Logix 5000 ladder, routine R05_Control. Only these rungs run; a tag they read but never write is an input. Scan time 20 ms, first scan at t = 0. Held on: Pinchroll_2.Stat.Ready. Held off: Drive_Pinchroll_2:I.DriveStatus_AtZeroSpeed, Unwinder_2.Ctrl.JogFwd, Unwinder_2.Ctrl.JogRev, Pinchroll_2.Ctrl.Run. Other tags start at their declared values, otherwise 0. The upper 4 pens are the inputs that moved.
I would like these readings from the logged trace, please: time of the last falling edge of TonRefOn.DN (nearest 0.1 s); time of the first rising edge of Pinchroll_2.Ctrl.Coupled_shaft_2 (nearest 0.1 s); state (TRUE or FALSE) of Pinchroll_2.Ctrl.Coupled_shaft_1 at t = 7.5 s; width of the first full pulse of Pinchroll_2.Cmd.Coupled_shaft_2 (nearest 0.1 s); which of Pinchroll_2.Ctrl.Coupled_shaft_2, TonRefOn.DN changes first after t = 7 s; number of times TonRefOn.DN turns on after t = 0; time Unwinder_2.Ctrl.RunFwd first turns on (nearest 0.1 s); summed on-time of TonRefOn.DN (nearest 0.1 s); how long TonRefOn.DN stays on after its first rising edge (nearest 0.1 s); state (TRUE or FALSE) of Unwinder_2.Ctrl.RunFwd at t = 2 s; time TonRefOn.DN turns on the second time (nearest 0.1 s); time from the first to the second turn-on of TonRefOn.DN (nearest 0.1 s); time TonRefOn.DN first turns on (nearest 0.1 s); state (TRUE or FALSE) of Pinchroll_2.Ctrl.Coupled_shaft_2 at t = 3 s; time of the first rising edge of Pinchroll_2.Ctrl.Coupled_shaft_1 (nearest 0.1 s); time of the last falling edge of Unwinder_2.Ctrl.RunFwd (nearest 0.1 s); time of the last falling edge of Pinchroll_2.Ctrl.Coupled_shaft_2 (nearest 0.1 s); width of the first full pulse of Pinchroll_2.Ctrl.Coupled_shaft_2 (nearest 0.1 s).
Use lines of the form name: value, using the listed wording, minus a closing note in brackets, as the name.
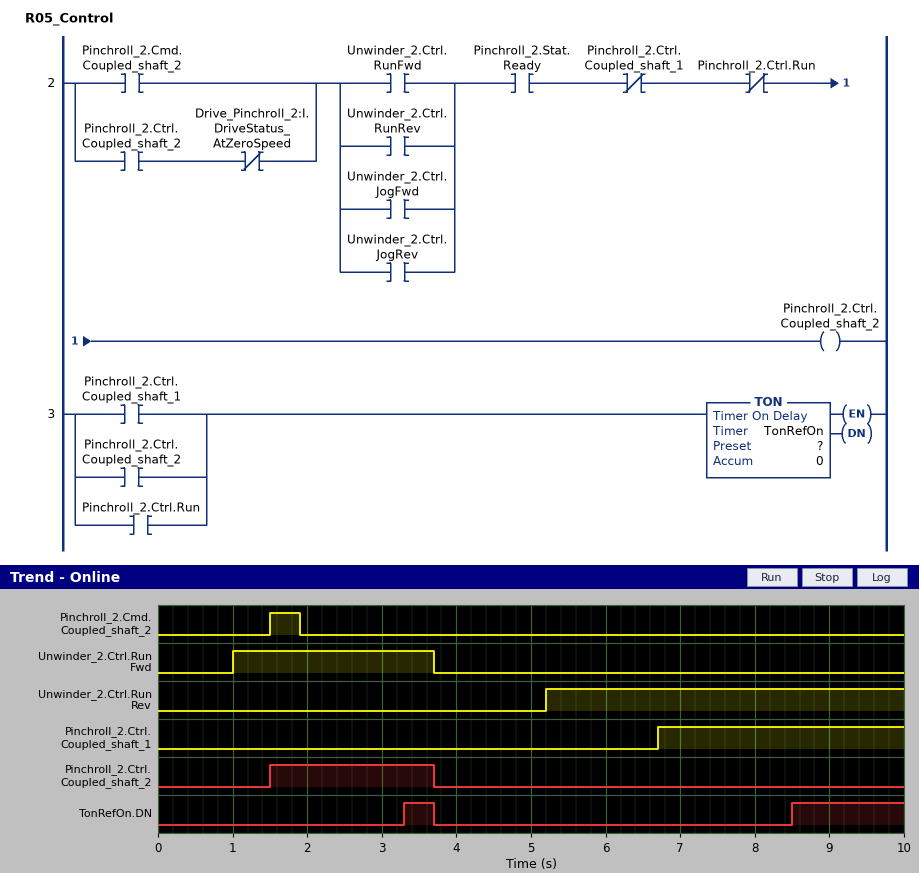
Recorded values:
time of the last falling edge of TonRefOn.DN: 3.7 s
time of the first rising edge of Pinchroll_2.Ctrl.Coupled_shaft_2: 1.5 s
state (TRUE or FALSE) of Pinchroll_2.Ctrl.Coupled_shaft_1 at t = 7.5 s: TRUE
width of the first full pulse of Pinchroll_2.Cmd.Coupled_shaft_2: 0.4 s
which of Pinchroll_2.Ctrl.Coupled_shaft_2, TonRefOn.DN changes first after t = 7 s: TonRefOn.DN
number of times TonRefOn.DN turns on after t = 0: 2
time Unwinder_2.Ctrl.RunFwd first turns on: 1.0 s
summed on-time of TonRefOn.DN: 1.9 s
how long TonRefOn.DN stays on after its first rising edge: 0.4 s
state (TRUE or FALSE) of Unwinder_2.Ctrl.RunFwd at t = 2 s: TRUE
time TonRefOn.DN turns on the second time: 8.5 s
time from the first to the second turn-on of TonRefOn.DN: 5.2 s
time TonRefOn.DN first turns on: 3.3 s
state (TRUE or FALSE) of Pinchroll_2.Ctrl.Coupled_shaft_2 at t = 3 s: TRUE
time of the first rising edge of Pinchroll_2.Ctrl.Coupled_shaft_1: 6.7 s
time of the last falling edge of Unwinder_2.Ctrl.RunFwd: 3.7 s
time of the last falling edge of Pinchroll_2.Ctrl.Coupled_shaft_2: 3.7 s
width of the first full pulse of Pinchroll_2.Ctrl.Coupled_shaft_2: 2.2 s
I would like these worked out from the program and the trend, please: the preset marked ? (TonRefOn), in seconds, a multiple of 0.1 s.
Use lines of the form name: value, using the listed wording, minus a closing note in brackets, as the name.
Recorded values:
the preset marked ? (TonRefOn), in seconds, a multiple of 0.1 s: 1.8 s
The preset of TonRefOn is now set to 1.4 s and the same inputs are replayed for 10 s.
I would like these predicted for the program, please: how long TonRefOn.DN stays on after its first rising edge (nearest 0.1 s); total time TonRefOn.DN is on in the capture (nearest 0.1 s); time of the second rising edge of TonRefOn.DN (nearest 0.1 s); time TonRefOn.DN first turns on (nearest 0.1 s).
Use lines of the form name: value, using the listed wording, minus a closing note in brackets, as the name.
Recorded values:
how long TonRefOn.DN stays on after its first rising edge: 0.8 s
total time TonRefOn.DN is on in the capture: 2.7 s
time of the second rising edge of TonRefOn.DN: 8.1 s
time TonRefOn.DN first turns on: 2.9 s
